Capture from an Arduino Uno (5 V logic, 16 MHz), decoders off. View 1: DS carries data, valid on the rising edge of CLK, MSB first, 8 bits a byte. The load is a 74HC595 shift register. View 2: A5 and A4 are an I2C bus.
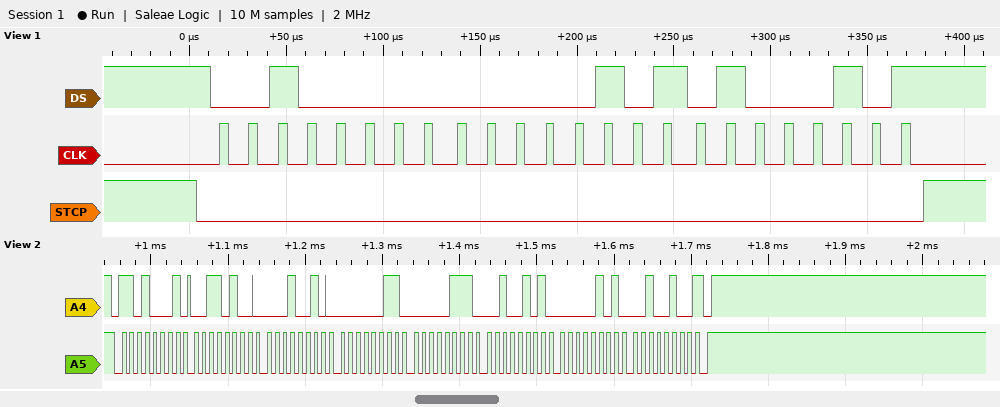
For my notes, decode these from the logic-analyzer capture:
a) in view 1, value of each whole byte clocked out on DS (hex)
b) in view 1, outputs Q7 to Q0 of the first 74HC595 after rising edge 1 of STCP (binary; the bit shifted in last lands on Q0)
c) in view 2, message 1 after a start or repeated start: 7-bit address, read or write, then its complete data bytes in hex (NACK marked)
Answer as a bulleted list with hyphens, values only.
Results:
- 0x20 0x05 0x45
- 01000101
- 0x68 read: 34 12 03 07 25 05 24 NACK
